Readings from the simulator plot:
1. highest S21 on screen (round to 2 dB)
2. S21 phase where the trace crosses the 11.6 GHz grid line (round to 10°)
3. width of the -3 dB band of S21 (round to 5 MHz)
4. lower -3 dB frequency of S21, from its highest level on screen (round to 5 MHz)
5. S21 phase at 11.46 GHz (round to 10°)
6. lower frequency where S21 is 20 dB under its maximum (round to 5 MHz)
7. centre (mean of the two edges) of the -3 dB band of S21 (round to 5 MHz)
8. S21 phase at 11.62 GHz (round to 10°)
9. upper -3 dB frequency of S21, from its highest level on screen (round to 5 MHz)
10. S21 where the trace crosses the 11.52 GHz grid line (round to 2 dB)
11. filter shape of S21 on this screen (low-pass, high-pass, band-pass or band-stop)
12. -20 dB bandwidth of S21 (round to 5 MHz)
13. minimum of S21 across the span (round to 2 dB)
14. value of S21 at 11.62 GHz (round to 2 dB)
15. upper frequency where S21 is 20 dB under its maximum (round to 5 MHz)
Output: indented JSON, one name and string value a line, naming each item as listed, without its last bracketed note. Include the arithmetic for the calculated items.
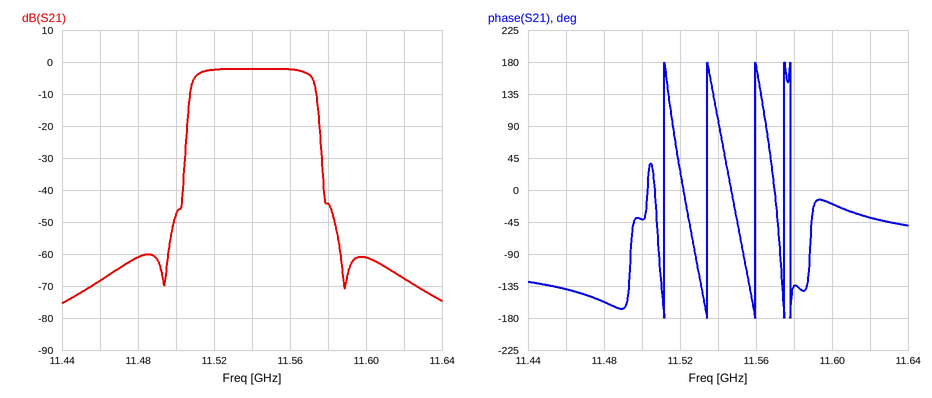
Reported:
{
  "highest S21 on screen": "-2 dB",
  "S21 phase where the trace crosses the 11.6 GHz grid line": "-20°",
  "width of the -3 dB band of S21": "11.570 GHz − 11.510 GHz = 60 MHz",
  "lower -3 dB frequency of S21, from its highest level on screen": "11.510 GHz",
  "S21 phase at 11.46 GHz": "-140°",
  "lower frequency where S21 is 20 dB under its maximum": "11.505 GHz",
  "centre (mean of the two edges) of the -3 dB band of S21": "11.540 GHz",
  "S21 phase at 11.62 GHz": "-40°",
  "upper -3 dB frequency of S21, from its highest level on screen": "11.570 GHz",
  "S21 where the trace crosses the 11.52 GHz grid line": "-2 dB",
  "filter shape of S21 on this screen": "band-pass",
  "-20 dB bandwidth of S21": "11.575 GHz − 11.505 GHz = 70 MHz",
  "minimum of S21 across the span": "-76 dB",
  "value of S21 at 11.62 GHz": "-68 dB",
  "upper frequency where S21 is 20 dB under its maximum": "11.575 GHz"
}
